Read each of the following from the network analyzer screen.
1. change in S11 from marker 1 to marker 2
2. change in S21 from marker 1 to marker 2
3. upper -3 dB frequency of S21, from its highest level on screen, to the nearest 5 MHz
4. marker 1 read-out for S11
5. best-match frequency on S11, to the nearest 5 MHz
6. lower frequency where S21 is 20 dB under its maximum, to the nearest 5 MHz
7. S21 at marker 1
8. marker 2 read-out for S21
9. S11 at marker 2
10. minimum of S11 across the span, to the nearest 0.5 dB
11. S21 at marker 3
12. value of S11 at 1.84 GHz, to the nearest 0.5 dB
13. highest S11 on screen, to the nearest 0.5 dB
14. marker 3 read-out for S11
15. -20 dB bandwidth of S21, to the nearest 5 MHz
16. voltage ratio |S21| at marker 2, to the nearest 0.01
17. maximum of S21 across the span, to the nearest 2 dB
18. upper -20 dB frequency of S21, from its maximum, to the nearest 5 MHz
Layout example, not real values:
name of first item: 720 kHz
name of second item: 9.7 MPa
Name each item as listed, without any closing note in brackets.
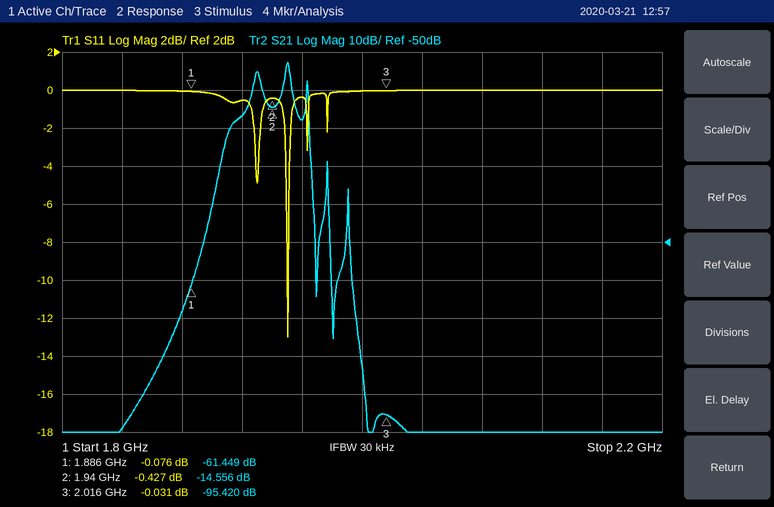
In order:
change in S11 from marker 1 to marker 2: -0.351 dB
change in S21 from marker 1 to marker 2: 46.893 dB
upper -3 dB frequency of S21, from its highest level on screen, to the nearest 5 MHz: 1.950 GHz
marker 1 read-out for S11: -0.076 dB
best-match frequency on S11, to the nearest 5 MHz: 1.950 GHz
lower frequency where S21 is 20 dB under its maximum, to the nearest 5 MHz: 1.910 GHz
S21 at marker 1: -61.449 dB
marker 2 read-out for S21: -14.556 dB
S11 at marker 2: -0.427 dB
minimum of S11 across the span, to the nearest 0.5 dB: -13.0 dB
S21 at marker 3: -95.420 dB
value of S11 at 1.84 GHz, to the nearest 0.5 dB: 0.0 dB
highest S11 on screen, to the nearest 0.5 dB: 0.0 dB
marker 3 read-out for S11: -0.031 dB
-20 dB bandwidth of S21, to the nearest 5 MHz: 55 MHz
voltage ratio |S21| at marker 2, to the nearest 0.01: 0.19
maximum of S21 across the span, to the nearest 2 dB: -2 dB
upper -20 dB frequency of S21, from its maximum, to the nearest 5 MHz: 1.965 GHz
